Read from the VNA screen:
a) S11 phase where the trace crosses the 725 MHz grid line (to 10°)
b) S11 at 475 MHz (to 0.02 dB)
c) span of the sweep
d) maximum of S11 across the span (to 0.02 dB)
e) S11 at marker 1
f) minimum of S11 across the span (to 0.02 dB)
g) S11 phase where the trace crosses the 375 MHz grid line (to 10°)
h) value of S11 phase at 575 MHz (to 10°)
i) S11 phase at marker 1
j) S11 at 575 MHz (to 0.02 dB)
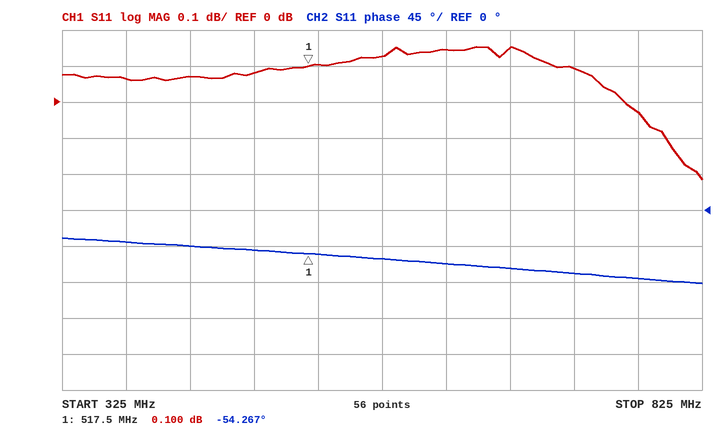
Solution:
-80°
0.08 dB
500 MHz
0.16 dB
0.100 dB
-0.22 dB
-40°
-60°
-54.267°
0.12 dB
